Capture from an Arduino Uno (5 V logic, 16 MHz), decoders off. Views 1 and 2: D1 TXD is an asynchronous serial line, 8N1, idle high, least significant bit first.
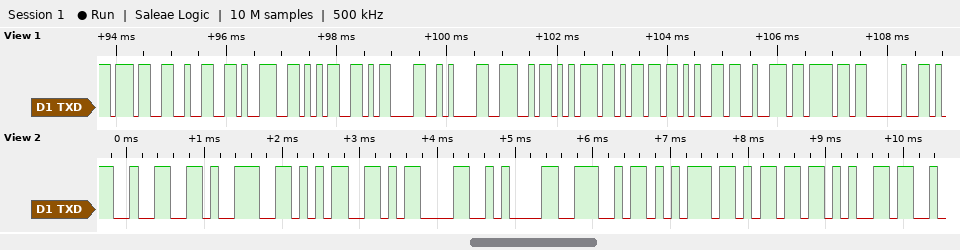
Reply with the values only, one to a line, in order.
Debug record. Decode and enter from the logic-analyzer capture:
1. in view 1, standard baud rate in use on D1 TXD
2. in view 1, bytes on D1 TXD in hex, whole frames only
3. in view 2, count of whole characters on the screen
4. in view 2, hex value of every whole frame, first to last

9600 baud
37 32 39 35 0D 0A 4E 75 6D 65 72 6F 20
9
32 39 35 0D 0A 4E 75 6D 65
